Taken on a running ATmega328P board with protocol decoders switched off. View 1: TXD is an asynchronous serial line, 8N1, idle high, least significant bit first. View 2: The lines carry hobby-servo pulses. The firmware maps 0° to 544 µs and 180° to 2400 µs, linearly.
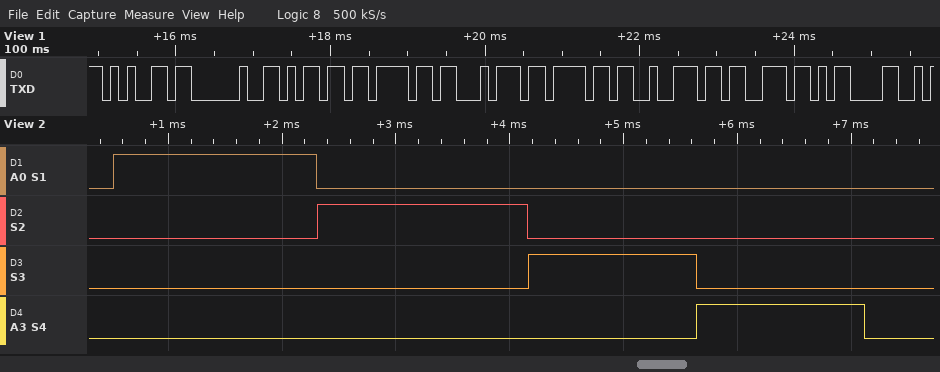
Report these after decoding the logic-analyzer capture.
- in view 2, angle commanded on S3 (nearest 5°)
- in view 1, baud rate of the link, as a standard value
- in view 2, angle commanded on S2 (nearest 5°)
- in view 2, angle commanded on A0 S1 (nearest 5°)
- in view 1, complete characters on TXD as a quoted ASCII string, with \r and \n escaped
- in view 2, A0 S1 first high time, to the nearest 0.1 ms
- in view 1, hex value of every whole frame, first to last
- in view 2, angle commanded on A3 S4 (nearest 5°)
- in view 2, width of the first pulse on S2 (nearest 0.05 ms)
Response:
90°
9600 baud
125°
120°
"e motors\r"
1.8 ms
65 20 6D 6F 74 6F 72 73 0D
90°
1.85 ms
